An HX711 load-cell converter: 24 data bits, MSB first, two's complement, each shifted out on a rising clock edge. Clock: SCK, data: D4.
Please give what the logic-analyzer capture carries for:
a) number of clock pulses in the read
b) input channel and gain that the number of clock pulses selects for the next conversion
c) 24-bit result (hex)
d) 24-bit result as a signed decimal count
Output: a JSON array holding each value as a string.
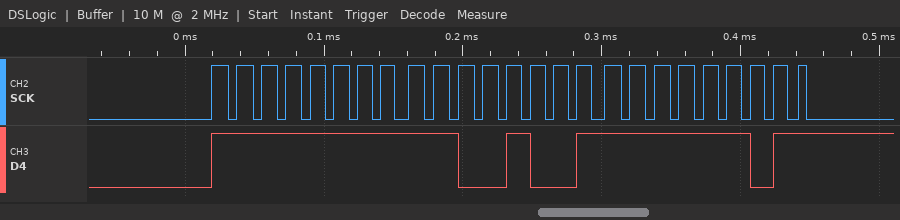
["25", "channel A, gain 128", "0xFFC9FD", "-13827"]
